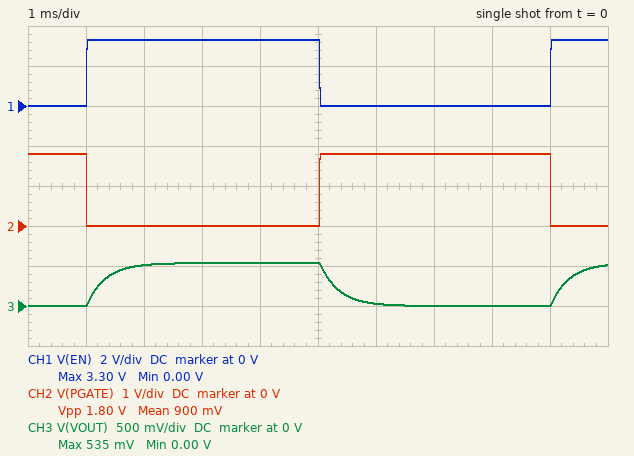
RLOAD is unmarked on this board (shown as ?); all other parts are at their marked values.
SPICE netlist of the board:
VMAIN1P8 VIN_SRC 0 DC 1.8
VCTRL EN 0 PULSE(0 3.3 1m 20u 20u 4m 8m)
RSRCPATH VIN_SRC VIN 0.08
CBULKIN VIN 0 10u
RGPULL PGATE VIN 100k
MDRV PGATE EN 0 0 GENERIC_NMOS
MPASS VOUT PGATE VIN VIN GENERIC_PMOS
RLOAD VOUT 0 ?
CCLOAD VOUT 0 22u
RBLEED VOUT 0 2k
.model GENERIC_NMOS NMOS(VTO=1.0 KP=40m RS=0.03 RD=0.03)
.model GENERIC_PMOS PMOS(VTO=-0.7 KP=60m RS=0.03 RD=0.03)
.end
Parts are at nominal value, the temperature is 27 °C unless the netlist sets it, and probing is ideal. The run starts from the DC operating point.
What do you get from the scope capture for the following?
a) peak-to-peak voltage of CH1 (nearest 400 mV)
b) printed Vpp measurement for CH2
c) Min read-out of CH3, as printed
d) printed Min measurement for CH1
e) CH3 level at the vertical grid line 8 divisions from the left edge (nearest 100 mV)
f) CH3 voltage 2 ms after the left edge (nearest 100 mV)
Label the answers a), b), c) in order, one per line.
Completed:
a) 3.2 V
b) 1.80 V
c) 0.00 V
d) 0.00 V
e) 0 V
f) 500 mV
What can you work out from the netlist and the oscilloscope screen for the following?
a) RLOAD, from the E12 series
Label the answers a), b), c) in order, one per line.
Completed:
a) 15 Ω
